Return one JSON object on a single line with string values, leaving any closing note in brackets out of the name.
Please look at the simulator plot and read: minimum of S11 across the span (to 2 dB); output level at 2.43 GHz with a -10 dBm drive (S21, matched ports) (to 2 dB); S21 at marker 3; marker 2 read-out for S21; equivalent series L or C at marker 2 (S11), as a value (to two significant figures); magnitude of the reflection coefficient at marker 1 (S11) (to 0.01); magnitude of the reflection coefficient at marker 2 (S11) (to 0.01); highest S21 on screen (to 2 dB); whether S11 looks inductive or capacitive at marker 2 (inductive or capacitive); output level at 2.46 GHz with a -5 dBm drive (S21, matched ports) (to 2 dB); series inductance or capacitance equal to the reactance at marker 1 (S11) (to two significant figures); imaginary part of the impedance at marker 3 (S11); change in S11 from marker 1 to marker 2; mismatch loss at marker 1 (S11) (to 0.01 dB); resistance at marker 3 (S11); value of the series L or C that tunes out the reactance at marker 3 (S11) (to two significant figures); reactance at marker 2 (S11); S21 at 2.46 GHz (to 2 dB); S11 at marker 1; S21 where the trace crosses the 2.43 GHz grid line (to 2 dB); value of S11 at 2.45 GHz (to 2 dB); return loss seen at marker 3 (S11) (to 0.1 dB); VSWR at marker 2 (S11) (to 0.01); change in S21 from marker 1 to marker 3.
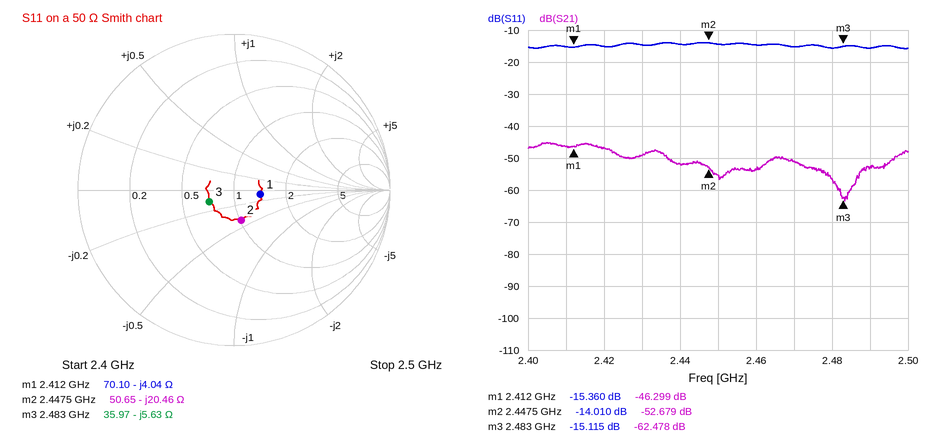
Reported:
{"minimum of S11 across the span": "-16 dB", "output level at 2.43 GHz with a -10 dBm drive (S21, matched ports)": "-60 dBm", "S21 at marker 3": "-62.478 dB", "marker 2 read-out for S21": "-52.679 dB", "equivalent series L or C at marker 2 (S11), as a value": "3.2 pF", "magnitude of the reflection coefficient at marker 1 (S11)": "0.17", "magnitude of the reflection coefficient at marker 2 (S11)": "0.20", "highest S21 on screen": "-46 dB", "whether S11 looks inductive or capacitive at marker 2": "capacitive", "output level at 2.46 GHz with a -5 dBm drive (S21, matched ports)": "-58 dBm", "series inductance or capacitance equal to the reactance at marker 1 (S11)": "16 pF", "imaginary part of the impedance at marker 3": "-5.63 Ω", "change in S11 from marker 1 to marker 2": "1.350 dB", "mismatch loss at marker 1 (S11)": "0.13 dB", "resistance at marker 3": "35.97 Ω", "value of the series L or C that tunes out the reactance at marker 3 (S11)": "360 pH", "reactance at marker 2": "-20.46 Ω", "S21 at 2.46 GHz": "-54 dB", "S11 at marker 1": "-15.360 dB", "S21 where the trace crosses the 2.43 GHz grid line": "-50 dB", "value of S11 at 2.45 GHz": "-14 dB", "return loss seen at marker 3 (S11)": "15.1 dB", "VSWR at marker 2 (S11)": "1.50", "change in S21 from marker 1 to marker 3": "-16.179 dB"}
